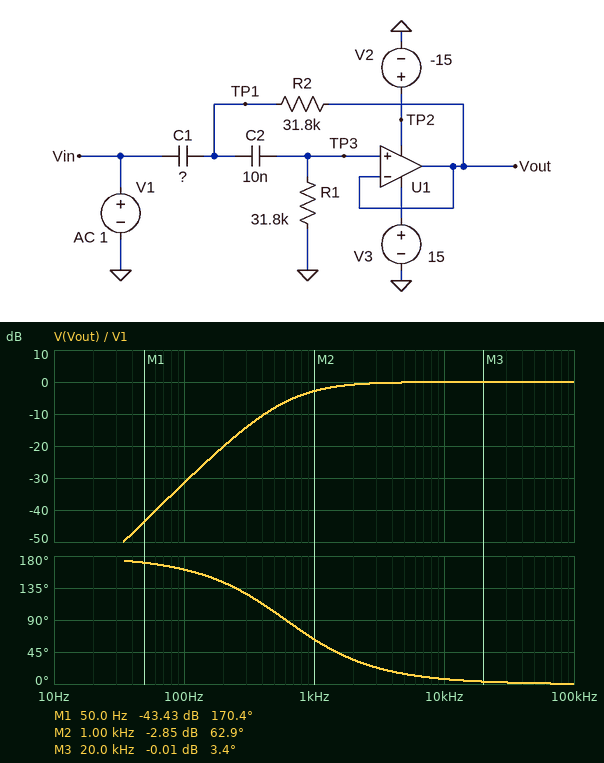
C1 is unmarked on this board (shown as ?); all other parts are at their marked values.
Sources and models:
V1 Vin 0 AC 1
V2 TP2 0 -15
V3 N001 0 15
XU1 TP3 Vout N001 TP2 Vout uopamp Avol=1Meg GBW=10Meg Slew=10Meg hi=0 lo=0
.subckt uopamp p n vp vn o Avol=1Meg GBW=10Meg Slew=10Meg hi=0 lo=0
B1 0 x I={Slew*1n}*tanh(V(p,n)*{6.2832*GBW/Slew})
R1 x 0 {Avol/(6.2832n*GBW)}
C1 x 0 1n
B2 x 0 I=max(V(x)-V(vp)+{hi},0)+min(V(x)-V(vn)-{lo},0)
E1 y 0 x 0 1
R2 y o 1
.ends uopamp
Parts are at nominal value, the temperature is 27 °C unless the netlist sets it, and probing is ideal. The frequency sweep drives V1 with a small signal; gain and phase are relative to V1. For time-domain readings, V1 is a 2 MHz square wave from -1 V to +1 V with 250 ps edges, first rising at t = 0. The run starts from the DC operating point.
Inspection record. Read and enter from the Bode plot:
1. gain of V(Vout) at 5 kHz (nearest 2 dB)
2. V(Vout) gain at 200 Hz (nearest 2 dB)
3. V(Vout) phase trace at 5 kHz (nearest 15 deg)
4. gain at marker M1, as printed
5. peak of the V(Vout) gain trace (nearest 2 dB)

0 dB
-20 dB
15 deg
-43.43 dB
0 dB
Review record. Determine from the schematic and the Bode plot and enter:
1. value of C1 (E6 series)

6.8 nF
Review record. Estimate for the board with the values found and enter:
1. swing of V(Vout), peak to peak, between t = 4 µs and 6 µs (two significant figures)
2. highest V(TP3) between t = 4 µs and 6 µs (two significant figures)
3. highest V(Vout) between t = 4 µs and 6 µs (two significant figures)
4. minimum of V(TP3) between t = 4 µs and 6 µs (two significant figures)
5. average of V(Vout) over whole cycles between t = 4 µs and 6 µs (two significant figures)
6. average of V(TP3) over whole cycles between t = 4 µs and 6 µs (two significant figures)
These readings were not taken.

2.0 V
2.0 V
2.0 V
-47 mV
960 mV
960 mV
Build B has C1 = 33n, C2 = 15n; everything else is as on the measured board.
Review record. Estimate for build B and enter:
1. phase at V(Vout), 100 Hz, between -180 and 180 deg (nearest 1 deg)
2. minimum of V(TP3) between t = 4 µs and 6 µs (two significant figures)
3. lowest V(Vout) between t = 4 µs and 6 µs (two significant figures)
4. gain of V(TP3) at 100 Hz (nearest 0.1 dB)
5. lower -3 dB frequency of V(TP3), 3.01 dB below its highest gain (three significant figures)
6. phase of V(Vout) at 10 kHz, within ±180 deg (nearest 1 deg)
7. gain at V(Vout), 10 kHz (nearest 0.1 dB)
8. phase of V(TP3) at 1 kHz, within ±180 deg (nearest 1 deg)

130 deg
-18 mV
-15 mV
-16.0 dB
389 Hz
3 deg
0 dB
27 deg
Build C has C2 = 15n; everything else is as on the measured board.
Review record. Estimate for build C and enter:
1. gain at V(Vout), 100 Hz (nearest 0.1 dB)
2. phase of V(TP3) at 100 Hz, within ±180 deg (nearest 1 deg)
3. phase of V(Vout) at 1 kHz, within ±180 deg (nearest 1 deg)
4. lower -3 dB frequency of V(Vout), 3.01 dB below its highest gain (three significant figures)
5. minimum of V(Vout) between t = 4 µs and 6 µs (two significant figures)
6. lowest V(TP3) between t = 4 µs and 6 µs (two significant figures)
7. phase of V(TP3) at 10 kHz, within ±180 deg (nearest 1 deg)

-28.3 dB
156 deg
55 deg
857 Hz
-36 mV
-41 mV
6 deg
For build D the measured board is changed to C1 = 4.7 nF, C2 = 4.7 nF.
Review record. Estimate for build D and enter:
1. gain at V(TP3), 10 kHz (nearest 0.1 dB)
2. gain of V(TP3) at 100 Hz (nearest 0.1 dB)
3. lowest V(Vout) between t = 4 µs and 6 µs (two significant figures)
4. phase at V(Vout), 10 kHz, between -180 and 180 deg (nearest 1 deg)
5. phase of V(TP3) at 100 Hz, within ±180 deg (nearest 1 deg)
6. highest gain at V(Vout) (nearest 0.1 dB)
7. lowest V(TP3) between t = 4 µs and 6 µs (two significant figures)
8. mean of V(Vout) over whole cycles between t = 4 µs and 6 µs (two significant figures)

-0.1 dB
-41.2 dB
-74 mV
12 deg
169 deg
0 dB
-79 mV
940 mV
